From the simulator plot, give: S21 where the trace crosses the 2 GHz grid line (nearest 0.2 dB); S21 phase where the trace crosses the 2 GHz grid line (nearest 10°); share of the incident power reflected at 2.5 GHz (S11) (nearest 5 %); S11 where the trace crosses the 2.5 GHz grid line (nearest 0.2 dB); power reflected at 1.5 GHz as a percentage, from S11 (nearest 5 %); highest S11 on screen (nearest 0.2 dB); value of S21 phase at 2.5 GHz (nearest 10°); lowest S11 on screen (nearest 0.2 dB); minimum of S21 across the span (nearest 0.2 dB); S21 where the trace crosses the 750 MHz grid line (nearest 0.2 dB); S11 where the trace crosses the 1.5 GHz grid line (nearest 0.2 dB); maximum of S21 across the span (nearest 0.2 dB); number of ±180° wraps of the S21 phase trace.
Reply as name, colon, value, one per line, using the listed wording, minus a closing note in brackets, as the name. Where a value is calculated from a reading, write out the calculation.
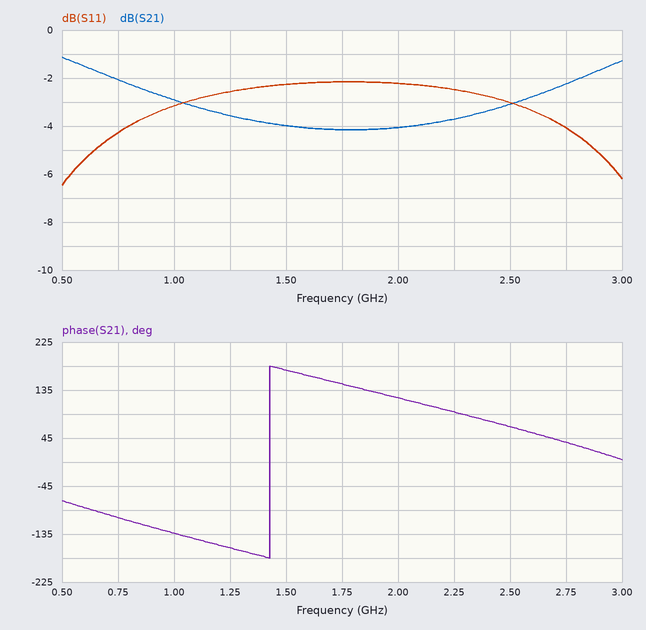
S21 where the trace crosses the 2 GHz grid line: -4.0 dB
S21 phase where the trace crosses the 2 GHz grid line: 120°
share of the incident power reflected at 2.5 GHz (S11): 10^(-3/10) ≈ 50 %
S11 where the trace crosses the 2.5 GHz grid line: -3.0 dB
power reflected at 1.5 GHz as a percentage, from S11: 10^(-2.2/10) ≈ 60 %
highest S11 on screen: -2.2 dB
value of S21 phase at 2.5 GHz: 70°
lowest S11 on screen: -6.4 dB
minimum of S21 across the span: -4.2 dB
S21 where the trace crosses the 750 MHz grid line: -2.0 dB
S11 where the trace crosses the 1.5 GHz grid line: -2.2 dB
maximum of S21 across the span: -1.2 dB
number of ±180° wraps of the S21 phase trace: 1
